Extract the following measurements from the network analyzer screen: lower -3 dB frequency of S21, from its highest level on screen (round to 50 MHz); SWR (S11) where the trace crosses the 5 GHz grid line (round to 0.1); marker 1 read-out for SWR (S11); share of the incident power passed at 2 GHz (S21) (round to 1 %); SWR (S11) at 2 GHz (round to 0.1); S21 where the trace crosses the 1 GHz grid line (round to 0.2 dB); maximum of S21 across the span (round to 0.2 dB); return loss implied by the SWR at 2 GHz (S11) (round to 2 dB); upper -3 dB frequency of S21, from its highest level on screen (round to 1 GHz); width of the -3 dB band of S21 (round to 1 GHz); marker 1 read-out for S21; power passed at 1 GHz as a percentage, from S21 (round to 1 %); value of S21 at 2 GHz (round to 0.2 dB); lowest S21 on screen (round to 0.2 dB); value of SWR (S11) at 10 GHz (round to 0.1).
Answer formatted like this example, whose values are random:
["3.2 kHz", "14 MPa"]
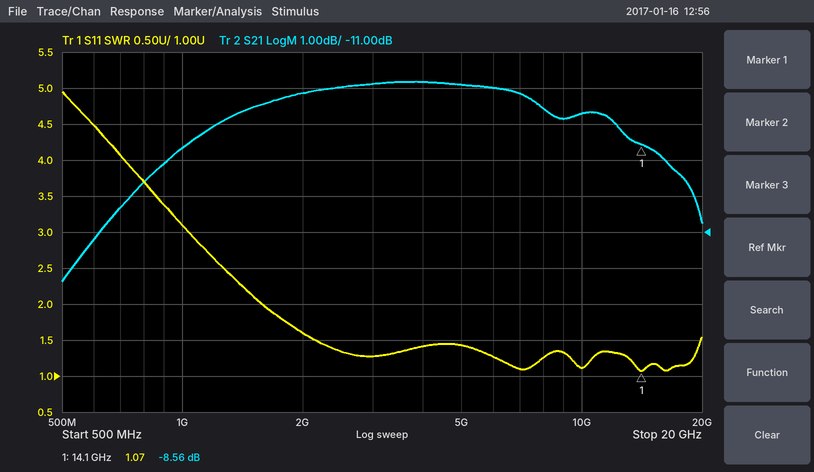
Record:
["750 MHz", "1.4", "1.07", "19 %", "1.6", "-8.6 dB", "-6.8 dB", "12 dB", "19 GHz", "18 GHz", "-8.56 dB", "14 %", "-7.2 dB", "-12.4 dB", "1.1"]
